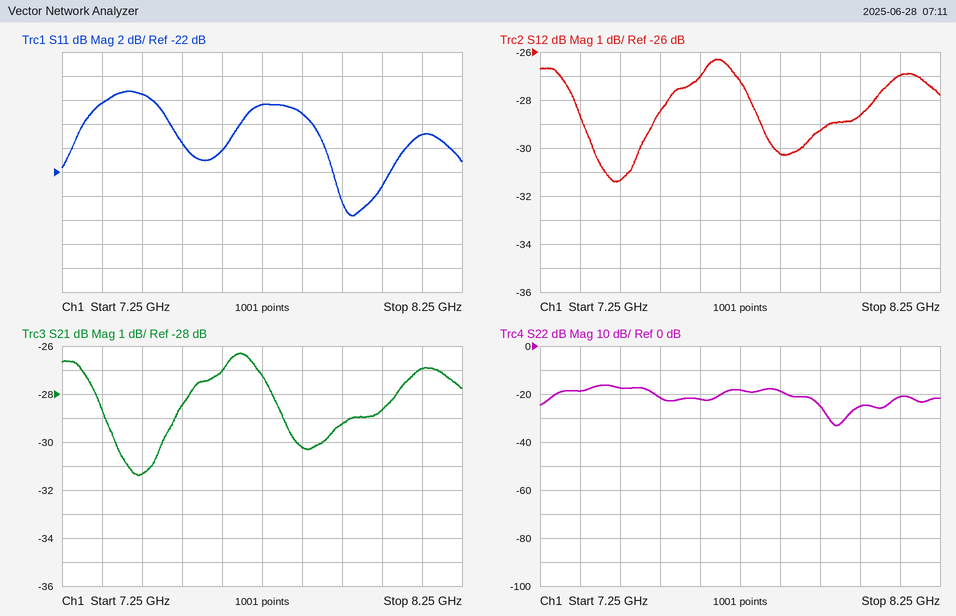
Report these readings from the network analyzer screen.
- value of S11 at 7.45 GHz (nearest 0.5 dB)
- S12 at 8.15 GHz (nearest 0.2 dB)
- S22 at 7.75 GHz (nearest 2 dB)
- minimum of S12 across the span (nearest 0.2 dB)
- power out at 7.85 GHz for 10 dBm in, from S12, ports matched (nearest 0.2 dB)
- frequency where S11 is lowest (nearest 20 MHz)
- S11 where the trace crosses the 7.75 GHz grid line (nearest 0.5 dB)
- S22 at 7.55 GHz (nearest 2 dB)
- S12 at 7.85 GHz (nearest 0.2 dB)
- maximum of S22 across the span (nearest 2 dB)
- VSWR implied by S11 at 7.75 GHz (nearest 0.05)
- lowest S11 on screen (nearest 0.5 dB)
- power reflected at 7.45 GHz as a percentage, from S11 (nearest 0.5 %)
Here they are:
-15.5 dB
-27.0 dB
-18 dB
-31.4 dB
-20.2 dBm
7.98 GHz
-16.5 dB
-22 dB
-30.2 dB
-16 dB
1.35
-25.5 dB
3.0 %
